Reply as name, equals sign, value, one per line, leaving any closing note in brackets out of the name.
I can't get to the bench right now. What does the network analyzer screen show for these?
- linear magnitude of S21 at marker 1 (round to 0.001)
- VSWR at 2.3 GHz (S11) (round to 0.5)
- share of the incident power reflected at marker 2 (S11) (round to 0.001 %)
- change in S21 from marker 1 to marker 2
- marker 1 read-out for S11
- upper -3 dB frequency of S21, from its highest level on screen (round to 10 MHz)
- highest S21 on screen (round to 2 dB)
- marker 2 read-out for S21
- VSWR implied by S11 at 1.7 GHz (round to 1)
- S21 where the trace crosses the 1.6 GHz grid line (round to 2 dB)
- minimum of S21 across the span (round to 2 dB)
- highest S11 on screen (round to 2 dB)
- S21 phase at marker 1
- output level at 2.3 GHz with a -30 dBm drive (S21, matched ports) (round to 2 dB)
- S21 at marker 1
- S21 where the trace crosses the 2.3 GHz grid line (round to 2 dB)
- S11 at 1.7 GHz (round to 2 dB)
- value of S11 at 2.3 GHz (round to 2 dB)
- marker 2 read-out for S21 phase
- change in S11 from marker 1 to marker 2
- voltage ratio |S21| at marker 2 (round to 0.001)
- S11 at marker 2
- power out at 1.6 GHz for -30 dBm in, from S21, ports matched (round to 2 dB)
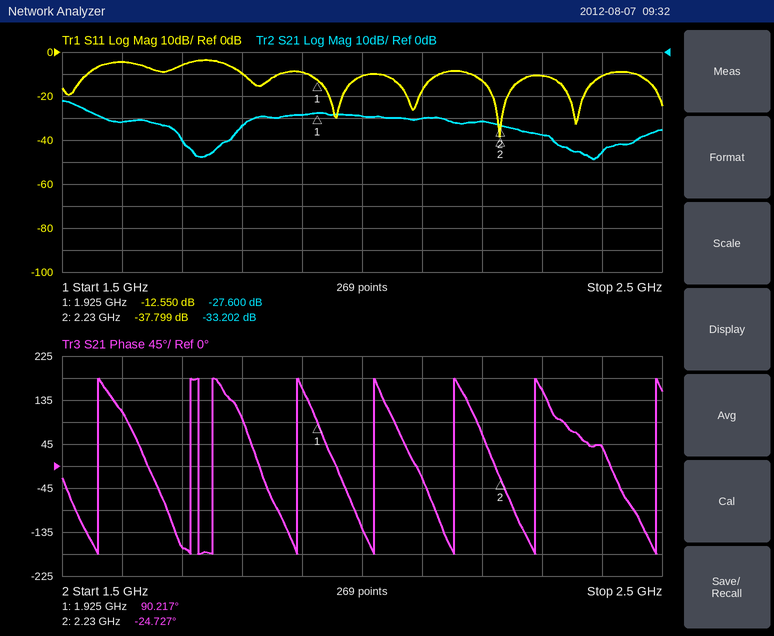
linear magnitude of S21 at marker 1 = 0.042
VSWR at 2.3 GHz (S11) = 2.0
share of the incident power reflected at marker 2 (S11) = 0.017 %
change in S21 from marker 1 to marker 2 = -5.602 dB
marker 1 read-out for S11 = -12.550 dB
upper -3 dB frequency of S21, from its highest level on screen = 1.53 GHz
highest S21 on screen = -22 dB
marker 2 read-out for S21 = -33.202 dB
VSWR implied by S11 at 1.7 GHz = 3
S21 where the trace crosses the 1.6 GHz grid line = -32 dB
minimum of S21 across the span = -48 dB
highest S11 on screen = -4 dB
S21 phase at marker 1 = 90.217°
output level at 2.3 GHz with a -30 dBm drive (S21, matched ports) = -68 dBm
S21 at marker 1 = -27.600 dB
S21 where the trace crosses the 2.3 GHz grid line = -38 dB
S11 at 1.7 GHz = -6 dB
value of S11 at 2.3 GHz = -10 dB
marker 2 read-out for S21 phase = -24.727°
change in S11 from marker 1 to marker 2 = -25.249 dB
voltage ratio |S21| at marker 2 = 0.022
S11 at marker 2 = -37.799 dB
power out at 1.6 GHz for -30 dBm in, from S21, ports matched = -62 dBm
